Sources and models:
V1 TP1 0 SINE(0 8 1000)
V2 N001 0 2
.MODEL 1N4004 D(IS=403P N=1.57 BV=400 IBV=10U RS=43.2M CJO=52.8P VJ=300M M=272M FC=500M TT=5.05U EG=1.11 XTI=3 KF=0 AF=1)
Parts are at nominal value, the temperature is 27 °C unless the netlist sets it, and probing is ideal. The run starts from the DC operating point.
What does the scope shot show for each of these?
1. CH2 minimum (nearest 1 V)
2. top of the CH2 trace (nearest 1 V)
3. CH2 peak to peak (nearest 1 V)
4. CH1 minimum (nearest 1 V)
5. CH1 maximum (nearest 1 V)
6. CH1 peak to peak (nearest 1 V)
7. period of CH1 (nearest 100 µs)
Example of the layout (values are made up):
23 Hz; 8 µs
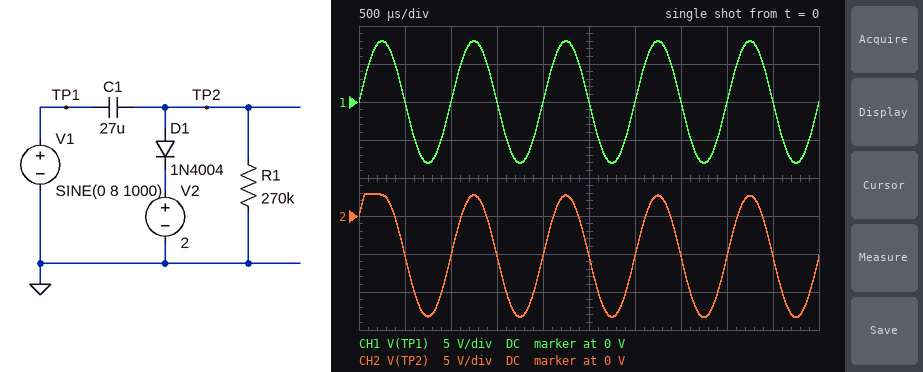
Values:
-13 V; 3 V; 16 V; -8 V; 8 V; 16 V; 1.0 ms
